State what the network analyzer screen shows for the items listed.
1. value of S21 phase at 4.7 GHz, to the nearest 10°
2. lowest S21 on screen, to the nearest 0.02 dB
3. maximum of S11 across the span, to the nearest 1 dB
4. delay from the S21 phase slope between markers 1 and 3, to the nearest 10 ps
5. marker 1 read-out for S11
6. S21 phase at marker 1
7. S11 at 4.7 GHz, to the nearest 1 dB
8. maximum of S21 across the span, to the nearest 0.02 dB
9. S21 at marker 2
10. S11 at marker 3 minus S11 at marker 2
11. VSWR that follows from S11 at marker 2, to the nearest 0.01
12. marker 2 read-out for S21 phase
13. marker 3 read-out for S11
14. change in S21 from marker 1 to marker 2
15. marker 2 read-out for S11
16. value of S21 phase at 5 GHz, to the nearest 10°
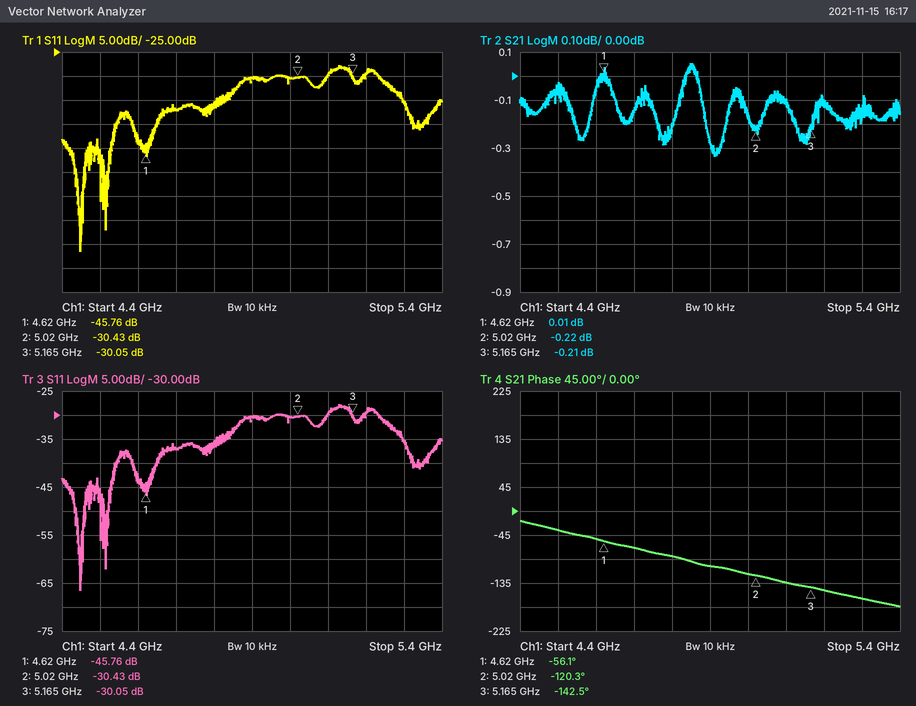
-70°
-0.34 dB
-28 dB
440 ps
-45.76 dB
-56.1°
-37 dB
0.06 dB
-0.22 dB
0.38 dB
1.06
-120.3°
-30.05 dB
-0.23 dB
-30.43 dB
-120°
